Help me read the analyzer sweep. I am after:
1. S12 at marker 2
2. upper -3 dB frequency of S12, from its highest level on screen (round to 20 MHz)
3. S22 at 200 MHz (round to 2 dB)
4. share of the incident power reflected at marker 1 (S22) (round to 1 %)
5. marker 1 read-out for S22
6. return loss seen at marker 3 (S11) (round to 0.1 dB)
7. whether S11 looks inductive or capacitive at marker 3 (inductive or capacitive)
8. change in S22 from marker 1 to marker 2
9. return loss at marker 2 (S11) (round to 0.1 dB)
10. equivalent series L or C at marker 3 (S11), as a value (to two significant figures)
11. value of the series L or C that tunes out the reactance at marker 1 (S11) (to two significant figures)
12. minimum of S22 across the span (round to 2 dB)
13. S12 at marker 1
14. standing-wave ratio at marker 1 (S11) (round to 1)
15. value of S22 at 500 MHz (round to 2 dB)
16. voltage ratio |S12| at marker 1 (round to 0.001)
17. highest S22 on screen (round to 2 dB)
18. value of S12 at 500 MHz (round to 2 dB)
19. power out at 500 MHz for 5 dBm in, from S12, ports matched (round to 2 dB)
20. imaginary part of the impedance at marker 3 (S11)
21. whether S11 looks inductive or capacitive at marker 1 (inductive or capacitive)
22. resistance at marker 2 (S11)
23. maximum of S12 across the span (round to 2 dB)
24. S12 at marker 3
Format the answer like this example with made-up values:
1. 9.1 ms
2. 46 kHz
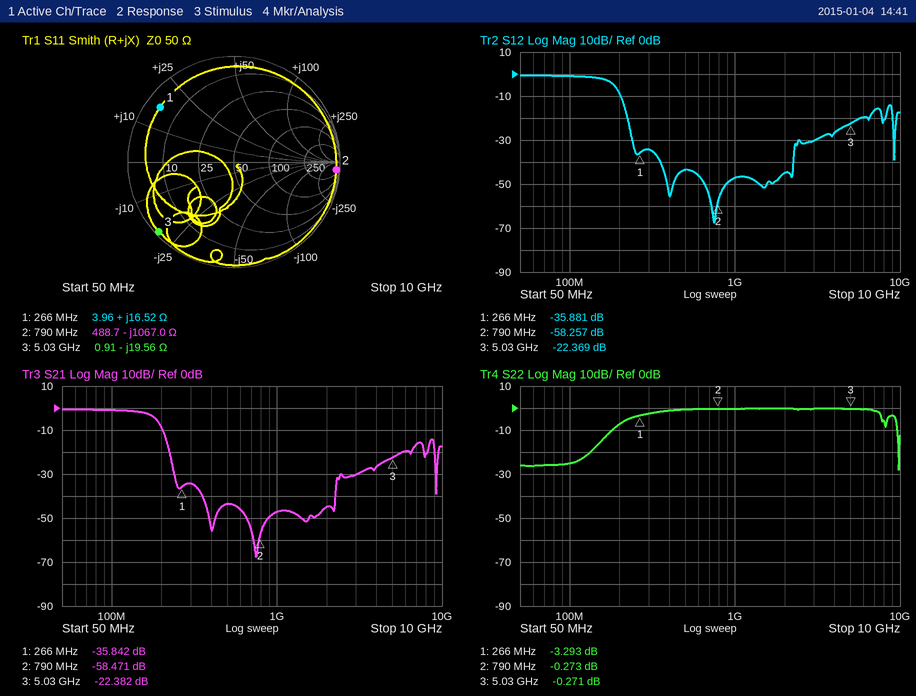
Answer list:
1. -58.257 dB
2. 180 MHz
3. -8 dB
4. 47 %
5. -3.293 dB
6. 0.3 dB
7. capacitive
8. 3.020 dB
9. 0.3 dB
10. 1.6 pF
11. 36 pF
12. -28 dB
13. -35.881 dB
14. 14
15. 0 dB
16. 0.016
17. 0 dB
18. -44 dB
19. -38 dBm
20. -19.56 Ω
21. inductive
22. 488.7 Ω
23. 0 dB
24. -22.369 dB
